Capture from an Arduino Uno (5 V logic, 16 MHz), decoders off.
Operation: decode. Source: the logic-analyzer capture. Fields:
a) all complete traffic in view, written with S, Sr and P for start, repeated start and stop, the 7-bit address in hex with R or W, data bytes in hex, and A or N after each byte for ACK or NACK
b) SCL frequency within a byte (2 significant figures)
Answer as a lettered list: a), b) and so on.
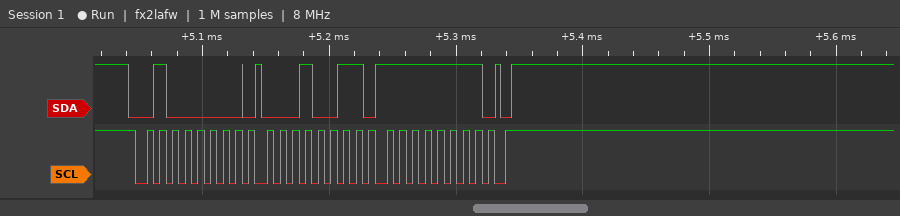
a) S 20W A 13 A FF A P
b) 100 kHz
